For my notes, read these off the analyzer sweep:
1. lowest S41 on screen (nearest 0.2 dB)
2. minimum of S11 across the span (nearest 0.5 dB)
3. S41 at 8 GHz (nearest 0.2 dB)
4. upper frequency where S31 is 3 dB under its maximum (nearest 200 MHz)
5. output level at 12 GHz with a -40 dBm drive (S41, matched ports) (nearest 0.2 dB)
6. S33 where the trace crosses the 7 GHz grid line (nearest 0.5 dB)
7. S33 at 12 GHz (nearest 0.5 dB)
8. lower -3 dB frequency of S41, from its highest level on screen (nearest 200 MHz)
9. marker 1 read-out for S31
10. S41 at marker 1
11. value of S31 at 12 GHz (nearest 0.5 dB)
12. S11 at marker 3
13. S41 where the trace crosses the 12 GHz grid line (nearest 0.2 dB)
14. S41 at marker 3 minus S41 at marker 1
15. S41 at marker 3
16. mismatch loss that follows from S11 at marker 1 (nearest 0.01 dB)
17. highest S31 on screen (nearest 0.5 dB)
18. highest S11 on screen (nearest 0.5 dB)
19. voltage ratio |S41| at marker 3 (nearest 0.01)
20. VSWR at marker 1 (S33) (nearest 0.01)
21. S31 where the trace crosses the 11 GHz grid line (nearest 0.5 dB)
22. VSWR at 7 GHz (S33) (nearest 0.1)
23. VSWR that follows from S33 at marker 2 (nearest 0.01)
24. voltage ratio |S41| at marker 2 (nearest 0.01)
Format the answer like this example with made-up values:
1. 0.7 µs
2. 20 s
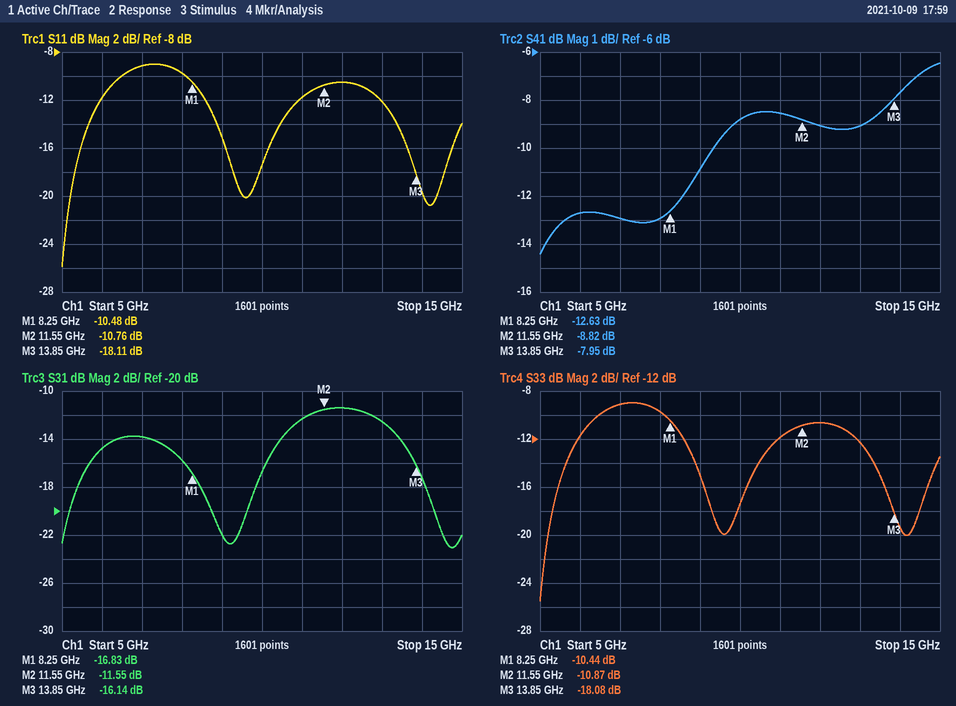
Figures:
1. -14.4 dB
2. -26.0 dB
3. -13.0 dB
4. 13.6 GHz
5. -49.0 dBm
6. -9.0 dB
7. -10.5 dB
8. 9.6 GHz
9. -16.83 dB
10. -12.63 dB
11. -11.5 dB
12. -18.11 dB
13. -9.0 dB
14. 4.68 dB
15. -7.95 dB
16. 0.41 dB
17. -11.5 dB
18. -9.0 dB
19. 0.40
20. 1.86
21. -12.5 dB
22. 2.1
23. 1.80
24. 0.36
